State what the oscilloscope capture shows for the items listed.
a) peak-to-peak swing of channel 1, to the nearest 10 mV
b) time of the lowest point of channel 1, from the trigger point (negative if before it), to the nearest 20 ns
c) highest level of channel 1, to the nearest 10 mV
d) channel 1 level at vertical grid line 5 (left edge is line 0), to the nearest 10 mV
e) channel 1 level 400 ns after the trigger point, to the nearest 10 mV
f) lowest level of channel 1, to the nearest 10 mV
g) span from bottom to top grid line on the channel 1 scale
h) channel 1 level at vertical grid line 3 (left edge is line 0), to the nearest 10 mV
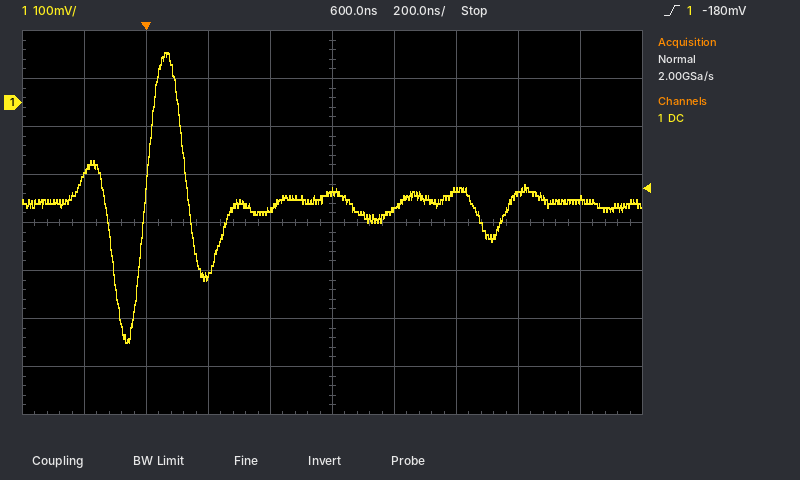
600 mV
-60 ns
100 mV
-190 mV
-220 mV
-500 mV
800 mV
-360 mV
